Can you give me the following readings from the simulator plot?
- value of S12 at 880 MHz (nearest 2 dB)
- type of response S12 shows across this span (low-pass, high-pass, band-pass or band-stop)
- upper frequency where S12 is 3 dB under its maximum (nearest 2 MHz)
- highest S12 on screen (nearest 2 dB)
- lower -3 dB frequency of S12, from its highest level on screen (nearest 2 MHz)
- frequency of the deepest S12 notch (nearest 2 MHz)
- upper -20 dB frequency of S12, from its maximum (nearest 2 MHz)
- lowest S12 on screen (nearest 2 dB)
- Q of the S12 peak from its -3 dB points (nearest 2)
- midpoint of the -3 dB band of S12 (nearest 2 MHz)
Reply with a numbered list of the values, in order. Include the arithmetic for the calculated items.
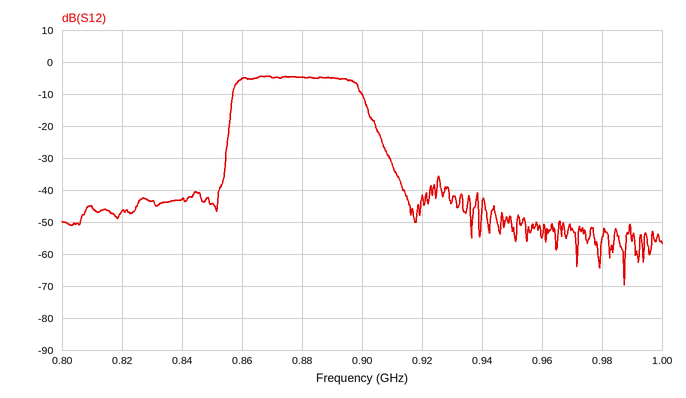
1. -4 dB
2. band-pass
3. 898 MHz
4. -4 dB
5. 858 MHz
6. 988 MHz
7. 906 MHz
8. -70 dB
9. 878 MHz / 40 MHz ≈ 22
10. 878 MHz
